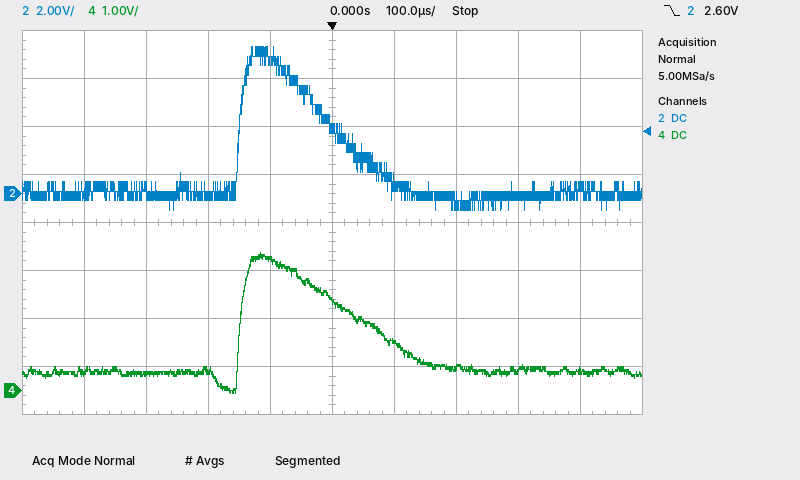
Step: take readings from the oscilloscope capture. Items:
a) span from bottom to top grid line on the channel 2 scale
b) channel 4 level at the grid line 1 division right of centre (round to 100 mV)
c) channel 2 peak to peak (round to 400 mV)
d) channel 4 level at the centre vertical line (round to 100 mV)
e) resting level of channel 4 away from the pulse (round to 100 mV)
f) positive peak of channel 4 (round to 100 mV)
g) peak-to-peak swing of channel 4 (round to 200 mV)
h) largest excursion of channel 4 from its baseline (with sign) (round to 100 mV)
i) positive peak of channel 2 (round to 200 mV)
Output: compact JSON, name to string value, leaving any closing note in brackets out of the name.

{"span from bottom to top grid line on the channel 2 scale": "16 V", "channel 4 level at the grid line 1 division right of centre": "1.0 V", "channel 2 peak to peak": "6.8 V", "channel 4 level at the centre vertical line": "1.9 V", "resting level of channel 4 away from the pulse": "400 mV", "positive peak of channel 4": "2.9 V", "peak-to-peak swing of channel 4": "3.0 V", "largest excursion of channel 4 from its baseline (with sign)": "+2.5 V", "positive peak of channel 2": "6.2 V"}
